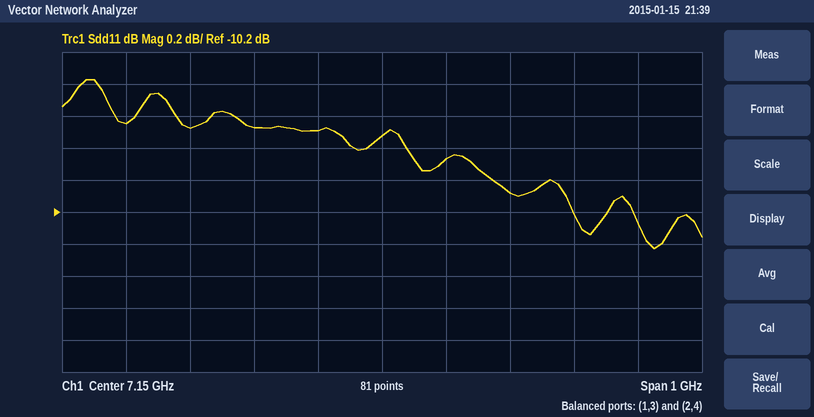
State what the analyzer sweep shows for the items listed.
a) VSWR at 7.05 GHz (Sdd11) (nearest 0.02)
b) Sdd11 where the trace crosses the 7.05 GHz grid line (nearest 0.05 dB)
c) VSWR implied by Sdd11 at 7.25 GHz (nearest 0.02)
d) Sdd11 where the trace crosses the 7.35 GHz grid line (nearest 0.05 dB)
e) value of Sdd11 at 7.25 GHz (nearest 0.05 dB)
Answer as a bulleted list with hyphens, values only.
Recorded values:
- 1.98
- -9.70 dB
- 1.94
- -10.10 dB
- -9.85 dB
